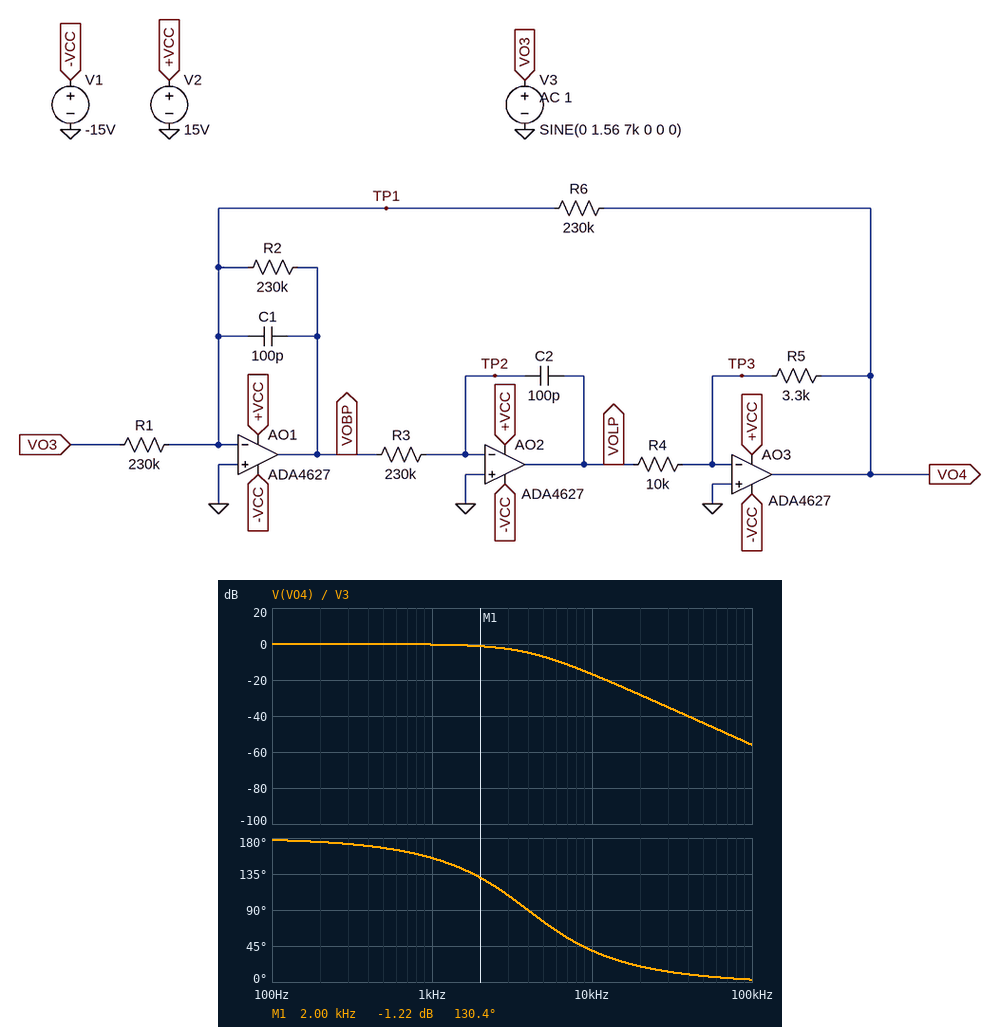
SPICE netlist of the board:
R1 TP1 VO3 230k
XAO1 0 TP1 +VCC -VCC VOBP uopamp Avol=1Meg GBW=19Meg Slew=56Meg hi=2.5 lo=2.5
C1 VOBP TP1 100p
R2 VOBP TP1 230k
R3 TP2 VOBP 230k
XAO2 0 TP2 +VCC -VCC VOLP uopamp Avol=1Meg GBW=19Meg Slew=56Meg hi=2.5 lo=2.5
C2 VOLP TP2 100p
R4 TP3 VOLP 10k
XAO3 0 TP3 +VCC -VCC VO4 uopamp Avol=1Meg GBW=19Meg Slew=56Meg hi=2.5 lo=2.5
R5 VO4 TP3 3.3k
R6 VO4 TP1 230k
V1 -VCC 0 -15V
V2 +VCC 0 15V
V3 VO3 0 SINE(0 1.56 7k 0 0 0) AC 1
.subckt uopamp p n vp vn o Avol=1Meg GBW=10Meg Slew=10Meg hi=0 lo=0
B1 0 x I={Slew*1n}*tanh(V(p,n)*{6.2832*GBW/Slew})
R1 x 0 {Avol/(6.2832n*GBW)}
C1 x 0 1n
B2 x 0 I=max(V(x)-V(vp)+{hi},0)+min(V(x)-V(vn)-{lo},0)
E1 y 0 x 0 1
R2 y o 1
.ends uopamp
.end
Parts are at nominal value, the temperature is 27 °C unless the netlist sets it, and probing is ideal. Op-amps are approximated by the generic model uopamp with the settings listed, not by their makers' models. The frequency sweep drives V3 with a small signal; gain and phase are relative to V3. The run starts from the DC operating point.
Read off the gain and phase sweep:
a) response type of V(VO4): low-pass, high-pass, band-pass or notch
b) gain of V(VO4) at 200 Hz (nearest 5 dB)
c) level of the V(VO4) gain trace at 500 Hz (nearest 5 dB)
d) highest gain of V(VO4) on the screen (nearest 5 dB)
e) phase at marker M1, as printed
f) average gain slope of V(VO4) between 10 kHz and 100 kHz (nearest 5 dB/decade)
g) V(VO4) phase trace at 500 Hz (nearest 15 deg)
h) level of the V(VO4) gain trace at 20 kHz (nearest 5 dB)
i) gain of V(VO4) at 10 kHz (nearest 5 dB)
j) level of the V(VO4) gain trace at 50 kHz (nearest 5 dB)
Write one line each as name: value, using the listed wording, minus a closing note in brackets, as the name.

response type of V(VO4): low-pass, high-pass, band-pass or notch: low-pass
gain of V(VO4) at 200 Hz: 0 dB
level of the V(VO4) gain trace at 500 Hz: 0 dB
highest gain of V(VO4) on the screen: 0 dB
phase at marker M1, as printed: 130.4 deg
average gain slope of V(VO4) between 10 kHz and 100 kHz: -40 dB/decade
V(VO4) phase trace at 500 Hz: 165 deg
level of the V(VO4) gain trace at 20 kHz: -30 dB
gain of V(VO4) at 10 kHz: -15 dB
level of the V(VO4) gain trace at 50 kHz: -45 dB
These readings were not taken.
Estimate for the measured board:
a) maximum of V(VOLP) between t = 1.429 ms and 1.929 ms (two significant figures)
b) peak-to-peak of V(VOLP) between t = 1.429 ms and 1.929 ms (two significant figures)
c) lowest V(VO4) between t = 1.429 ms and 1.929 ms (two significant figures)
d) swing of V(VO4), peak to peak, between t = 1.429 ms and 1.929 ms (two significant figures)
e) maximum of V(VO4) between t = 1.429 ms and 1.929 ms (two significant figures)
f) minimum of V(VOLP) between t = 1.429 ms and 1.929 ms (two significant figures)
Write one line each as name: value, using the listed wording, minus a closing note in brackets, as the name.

maximum of V(VOLP) between t = 1.429 ms and 1.929 ms: 1.3 V
peak-to-peak of V(VOLP) between t = 1.429 ms and 1.929 ms: 2.5 V
lowest V(VO4) between t = 1.429 ms and 1.929 ms: -420 mV
swing of V(VO4), peak to peak, between t = 1.429 ms and 1.929 ms: 840 mV
maximum of V(VO4) between t = 1.429 ms and 1.929 ms: 420 mV
minimum of V(VOLP) between t = 1.429 ms and 1.929 ms: -1.3 V
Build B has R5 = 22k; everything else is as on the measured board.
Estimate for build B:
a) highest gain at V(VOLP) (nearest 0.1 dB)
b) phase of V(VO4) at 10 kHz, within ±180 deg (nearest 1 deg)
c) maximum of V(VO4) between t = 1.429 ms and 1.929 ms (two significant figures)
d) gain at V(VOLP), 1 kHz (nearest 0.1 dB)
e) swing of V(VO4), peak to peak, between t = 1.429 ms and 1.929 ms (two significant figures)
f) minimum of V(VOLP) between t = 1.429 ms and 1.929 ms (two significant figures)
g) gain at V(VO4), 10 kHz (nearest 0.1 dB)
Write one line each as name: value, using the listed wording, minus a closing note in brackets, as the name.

highest gain at V(VOLP): -2.9 dB
phase of V(VO4) at 10 kHz, within ±180 deg: 94 deg
maximum of V(VO4) between t = 1.429 ms and 1.929 ms: 2.2 V
gain at V(VOLP), 1 kHz: -6.8 dB
swing of V(VO4), peak to peak, between t = 1.429 ms and 1.929 ms: 4.4 V
minimum of V(VOLP) between t = 1.429 ms and 1.929 ms: -1.0 V
gain at V(VO4), 10 kHz: 3.7 dB
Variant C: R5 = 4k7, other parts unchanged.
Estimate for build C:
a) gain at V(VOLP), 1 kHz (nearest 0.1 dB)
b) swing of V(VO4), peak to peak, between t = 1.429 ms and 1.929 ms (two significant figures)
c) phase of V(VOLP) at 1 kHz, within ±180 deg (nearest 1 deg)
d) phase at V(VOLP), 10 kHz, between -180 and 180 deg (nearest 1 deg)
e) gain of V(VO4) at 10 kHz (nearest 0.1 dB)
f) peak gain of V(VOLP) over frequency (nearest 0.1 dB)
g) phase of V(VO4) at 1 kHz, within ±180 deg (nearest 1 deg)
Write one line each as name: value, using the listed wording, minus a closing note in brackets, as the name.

gain at V(VOLP), 1 kHz: 6.5 dB
swing of V(VO4), peak to peak, between t = 1.429 ms and 1.929 ms: 1.3 V
phase of V(VOLP) at 1 kHz, within ±180 deg: -18 deg
phase at V(VOLP), 10 kHz, between -180 and 180 deg: -138 deg
gain of V(VO4) at 10 kHz: -13.3 dB
peak gain of V(VOLP) over frequency: 6.6 dB
phase of V(VO4) at 1 kHz, within ±180 deg: 162 deg
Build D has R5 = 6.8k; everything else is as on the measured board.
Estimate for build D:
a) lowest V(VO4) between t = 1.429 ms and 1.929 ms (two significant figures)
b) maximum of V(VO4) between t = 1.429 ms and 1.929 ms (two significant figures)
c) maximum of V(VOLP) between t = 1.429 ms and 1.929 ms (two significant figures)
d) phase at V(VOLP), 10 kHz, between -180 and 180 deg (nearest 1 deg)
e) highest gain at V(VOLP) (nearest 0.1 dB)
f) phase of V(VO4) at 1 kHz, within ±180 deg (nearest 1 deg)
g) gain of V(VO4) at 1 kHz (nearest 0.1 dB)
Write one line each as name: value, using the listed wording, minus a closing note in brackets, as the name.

lowest V(VO4) between t = 1.429 ms and 1.929 ms: -990 mV
maximum of V(VO4) between t = 1.429 ms and 1.929 ms: 990 mV
maximum of V(VOLP) between t = 1.429 ms and 1.929 ms: 1.5 V
phase at V(VOLP), 10 kHz, between -180 and 180 deg: -134 deg
highest gain at V(VOLP): 3.7 dB
phase of V(VO4) at 1 kHz, within ±180 deg: 168 deg
gain of V(VO4) at 1 kHz: 0.1 dB
